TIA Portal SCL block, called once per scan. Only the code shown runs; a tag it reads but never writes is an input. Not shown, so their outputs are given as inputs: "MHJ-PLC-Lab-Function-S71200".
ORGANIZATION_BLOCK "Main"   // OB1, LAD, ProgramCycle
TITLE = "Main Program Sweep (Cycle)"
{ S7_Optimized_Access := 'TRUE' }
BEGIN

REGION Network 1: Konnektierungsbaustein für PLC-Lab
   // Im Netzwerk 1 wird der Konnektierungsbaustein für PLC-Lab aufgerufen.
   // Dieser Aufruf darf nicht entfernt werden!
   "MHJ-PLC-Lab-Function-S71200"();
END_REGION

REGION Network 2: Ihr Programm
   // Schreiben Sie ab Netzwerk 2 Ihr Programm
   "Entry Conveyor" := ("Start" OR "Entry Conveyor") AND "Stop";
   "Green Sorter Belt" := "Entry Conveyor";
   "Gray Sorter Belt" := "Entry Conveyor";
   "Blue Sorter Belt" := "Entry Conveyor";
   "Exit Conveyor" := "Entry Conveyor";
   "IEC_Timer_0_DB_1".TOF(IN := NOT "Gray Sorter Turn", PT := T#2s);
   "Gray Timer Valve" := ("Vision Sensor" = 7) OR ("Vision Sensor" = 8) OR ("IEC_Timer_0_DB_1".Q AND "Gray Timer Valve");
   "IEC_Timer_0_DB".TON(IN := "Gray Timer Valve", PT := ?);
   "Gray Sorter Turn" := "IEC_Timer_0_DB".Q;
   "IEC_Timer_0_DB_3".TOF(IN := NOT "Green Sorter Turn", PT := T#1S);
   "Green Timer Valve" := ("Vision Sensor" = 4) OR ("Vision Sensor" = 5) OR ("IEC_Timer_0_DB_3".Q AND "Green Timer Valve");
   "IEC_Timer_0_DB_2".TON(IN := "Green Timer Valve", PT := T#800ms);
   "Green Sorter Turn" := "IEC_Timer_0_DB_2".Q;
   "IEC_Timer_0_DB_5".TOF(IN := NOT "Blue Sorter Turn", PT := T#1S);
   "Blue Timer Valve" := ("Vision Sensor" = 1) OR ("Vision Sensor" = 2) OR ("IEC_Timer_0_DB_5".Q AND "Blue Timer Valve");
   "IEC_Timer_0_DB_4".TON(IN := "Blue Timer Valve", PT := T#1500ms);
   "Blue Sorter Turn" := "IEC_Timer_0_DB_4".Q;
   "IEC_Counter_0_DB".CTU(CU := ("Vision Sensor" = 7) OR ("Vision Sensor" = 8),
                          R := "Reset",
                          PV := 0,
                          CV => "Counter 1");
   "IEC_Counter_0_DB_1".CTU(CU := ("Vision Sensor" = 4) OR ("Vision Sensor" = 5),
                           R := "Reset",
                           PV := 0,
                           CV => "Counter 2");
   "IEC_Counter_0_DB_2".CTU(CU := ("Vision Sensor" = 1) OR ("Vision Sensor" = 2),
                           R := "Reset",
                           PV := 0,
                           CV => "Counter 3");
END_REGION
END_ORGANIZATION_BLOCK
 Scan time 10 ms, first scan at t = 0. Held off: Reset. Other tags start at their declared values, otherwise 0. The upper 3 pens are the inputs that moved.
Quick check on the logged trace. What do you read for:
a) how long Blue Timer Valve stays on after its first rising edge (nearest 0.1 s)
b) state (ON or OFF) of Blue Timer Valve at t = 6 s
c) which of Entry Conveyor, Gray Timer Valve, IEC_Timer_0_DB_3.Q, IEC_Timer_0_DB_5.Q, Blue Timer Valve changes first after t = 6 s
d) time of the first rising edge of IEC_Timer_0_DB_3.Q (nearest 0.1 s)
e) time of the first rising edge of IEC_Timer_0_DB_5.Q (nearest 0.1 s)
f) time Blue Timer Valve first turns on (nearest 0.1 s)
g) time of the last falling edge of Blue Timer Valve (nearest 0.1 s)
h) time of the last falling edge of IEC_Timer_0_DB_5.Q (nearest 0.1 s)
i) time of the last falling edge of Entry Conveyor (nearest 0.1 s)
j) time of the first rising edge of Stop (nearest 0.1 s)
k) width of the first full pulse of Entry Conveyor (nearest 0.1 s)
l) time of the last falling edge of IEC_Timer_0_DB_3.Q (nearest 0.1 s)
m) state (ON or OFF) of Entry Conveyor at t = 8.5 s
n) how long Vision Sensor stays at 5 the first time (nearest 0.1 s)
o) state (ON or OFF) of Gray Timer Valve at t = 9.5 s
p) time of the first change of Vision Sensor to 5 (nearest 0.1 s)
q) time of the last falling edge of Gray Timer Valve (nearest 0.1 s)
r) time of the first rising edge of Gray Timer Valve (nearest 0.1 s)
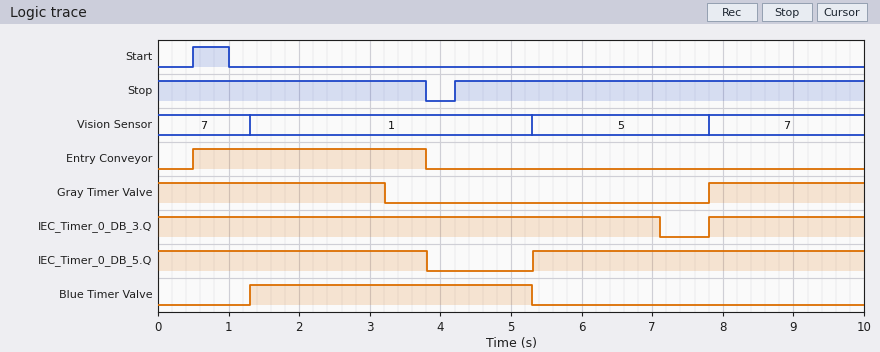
4.0 s
OFF
IEC_Timer_0_DB_3.Q
7.8 s
5.3 s
1.3 s
5.3 s
3.8 s
3.8 s
4.2 s
3.3 s
7.1 s
OFF
2.5 s
ON
5.3 s
3.2 s
7.8 s
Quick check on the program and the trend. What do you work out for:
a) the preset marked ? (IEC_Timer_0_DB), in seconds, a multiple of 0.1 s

1.2 s
